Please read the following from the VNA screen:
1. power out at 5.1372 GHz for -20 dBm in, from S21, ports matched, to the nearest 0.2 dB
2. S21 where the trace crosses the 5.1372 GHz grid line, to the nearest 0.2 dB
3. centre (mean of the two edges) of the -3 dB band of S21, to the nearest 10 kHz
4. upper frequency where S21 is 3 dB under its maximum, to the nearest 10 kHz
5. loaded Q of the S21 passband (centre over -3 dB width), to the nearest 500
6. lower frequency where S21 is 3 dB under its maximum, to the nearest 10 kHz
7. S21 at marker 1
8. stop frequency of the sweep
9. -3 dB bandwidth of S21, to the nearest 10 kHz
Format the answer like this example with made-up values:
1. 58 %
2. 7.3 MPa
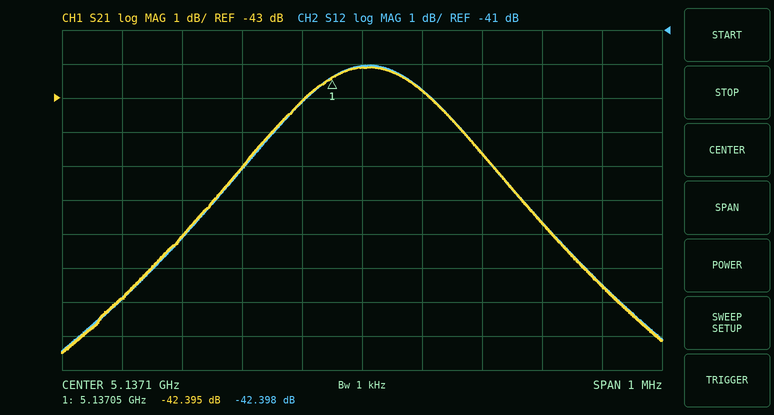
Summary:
1. -62.8 dBm
2. -42.8 dB
3. 5.13711 GHz
4. 5.13732 GHz
5. 12000
6. 5.13690 GHz
7. -42.395 dB
8. 5.1376 GHz
9. 420 kHz
